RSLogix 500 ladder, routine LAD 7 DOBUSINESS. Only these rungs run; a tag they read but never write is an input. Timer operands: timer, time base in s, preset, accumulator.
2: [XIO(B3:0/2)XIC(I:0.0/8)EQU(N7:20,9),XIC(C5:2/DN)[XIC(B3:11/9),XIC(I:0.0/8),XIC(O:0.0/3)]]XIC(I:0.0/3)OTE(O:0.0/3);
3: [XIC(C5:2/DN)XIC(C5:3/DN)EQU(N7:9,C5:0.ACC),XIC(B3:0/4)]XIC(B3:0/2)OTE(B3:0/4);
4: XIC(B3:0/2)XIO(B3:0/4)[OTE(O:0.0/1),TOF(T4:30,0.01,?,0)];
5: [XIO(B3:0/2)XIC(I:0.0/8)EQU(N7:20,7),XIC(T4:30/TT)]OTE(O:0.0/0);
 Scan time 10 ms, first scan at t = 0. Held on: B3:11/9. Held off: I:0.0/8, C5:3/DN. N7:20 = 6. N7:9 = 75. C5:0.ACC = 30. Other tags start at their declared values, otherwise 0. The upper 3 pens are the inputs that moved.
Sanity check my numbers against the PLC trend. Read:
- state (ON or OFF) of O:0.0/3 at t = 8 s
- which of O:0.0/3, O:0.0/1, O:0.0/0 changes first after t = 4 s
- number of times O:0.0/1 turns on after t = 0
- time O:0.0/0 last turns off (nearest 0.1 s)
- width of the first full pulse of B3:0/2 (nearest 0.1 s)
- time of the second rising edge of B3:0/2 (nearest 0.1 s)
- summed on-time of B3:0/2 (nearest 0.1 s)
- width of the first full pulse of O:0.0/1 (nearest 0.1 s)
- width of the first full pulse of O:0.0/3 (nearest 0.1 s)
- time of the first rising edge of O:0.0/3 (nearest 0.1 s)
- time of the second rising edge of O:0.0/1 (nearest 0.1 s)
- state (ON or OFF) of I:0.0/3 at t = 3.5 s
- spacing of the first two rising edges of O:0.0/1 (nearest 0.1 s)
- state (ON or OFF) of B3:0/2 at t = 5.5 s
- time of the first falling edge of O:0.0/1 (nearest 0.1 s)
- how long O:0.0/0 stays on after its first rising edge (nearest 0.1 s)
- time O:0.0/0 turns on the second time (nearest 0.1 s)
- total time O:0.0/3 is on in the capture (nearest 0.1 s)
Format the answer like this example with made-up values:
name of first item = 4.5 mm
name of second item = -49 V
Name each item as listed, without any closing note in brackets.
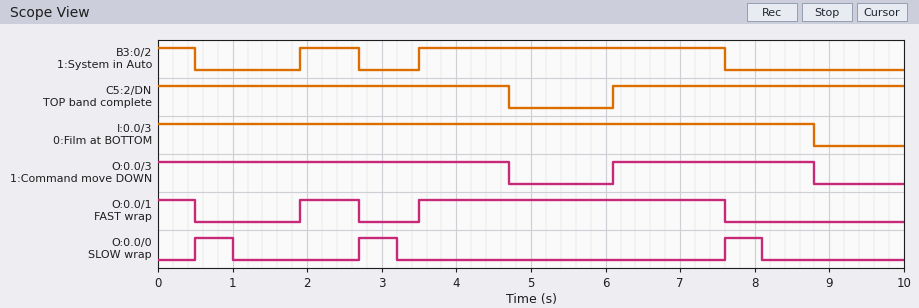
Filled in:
state (ON or OFF) of O:0.0/3 at t = 8 s = ON
which of O:0.0/3, O:0.0/1, O:0.0/0 changes first after t = 4 s = O:0.0/3
number of times O:0.0/1 turns on after t = 0 = 2
time O:0.0/0 last turns off = 8.1 s
width of the first full pulse of B3:0/2 = 0.8 s
time of the second rising edge of B3:0/2 = 3.5 s
summed on-time of B3:0/2 = 5.4 s
width of the first full pulse of O:0.0/1 = 0.8 s
width of the first full pulse of O:0.0/3 = 2.7 s
time of the first rising edge of O:0.0/3 = 6.1 s
time of the second rising edge of O:0.0/1 = 3.5 s
state (ON or OFF) of I:0.0/3 at t = 3.5 s = ON
spacing of the first two rising edges of O:0.0/1 = 1.6 s
state (ON or OFF) of B3:0/2 at t = 5.5 s = ON
time of the first falling edge of O:0.0/1 = 0.5 s
how long O:0.0/0 stays on after its first rising edge = 0.5 s
time O:0.0/0 turns on the second time = 2.7 s
total time O:0.0/3 is on in the capture = 7.4 s
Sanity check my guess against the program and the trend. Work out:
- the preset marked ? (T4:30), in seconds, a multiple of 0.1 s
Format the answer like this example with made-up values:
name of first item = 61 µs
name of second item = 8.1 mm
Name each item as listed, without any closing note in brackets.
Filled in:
the preset marked ? (T4:30), in seconds, a multiple of 0.1 s = 0.5 s
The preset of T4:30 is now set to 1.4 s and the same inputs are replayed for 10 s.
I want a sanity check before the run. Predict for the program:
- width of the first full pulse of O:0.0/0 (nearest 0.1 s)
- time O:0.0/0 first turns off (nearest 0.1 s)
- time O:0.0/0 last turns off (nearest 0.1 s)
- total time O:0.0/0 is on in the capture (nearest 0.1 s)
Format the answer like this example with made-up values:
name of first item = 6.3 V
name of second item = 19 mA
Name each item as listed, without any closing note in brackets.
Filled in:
width of the first full pulse of O:0.0/0 = 1.4 s
time O:0.0/0 first turns off = 1.9 s
time O:0.0/0 last turns off = 9.0 s
total time O:0.0/0 is on in the capture = 3.6 s
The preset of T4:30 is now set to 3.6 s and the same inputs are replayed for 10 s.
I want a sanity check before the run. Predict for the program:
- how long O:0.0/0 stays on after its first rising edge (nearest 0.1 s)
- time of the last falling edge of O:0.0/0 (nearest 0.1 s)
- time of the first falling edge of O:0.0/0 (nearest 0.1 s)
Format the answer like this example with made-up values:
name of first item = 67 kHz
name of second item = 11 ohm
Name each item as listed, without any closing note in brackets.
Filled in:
how long O:0.0/0 stays on after its first rising edge = 1.4 s
time of the last falling edge of O:0.0/0 = 3.5 s
time of the first falling edge of O:0.0/0 = 1.9 s
